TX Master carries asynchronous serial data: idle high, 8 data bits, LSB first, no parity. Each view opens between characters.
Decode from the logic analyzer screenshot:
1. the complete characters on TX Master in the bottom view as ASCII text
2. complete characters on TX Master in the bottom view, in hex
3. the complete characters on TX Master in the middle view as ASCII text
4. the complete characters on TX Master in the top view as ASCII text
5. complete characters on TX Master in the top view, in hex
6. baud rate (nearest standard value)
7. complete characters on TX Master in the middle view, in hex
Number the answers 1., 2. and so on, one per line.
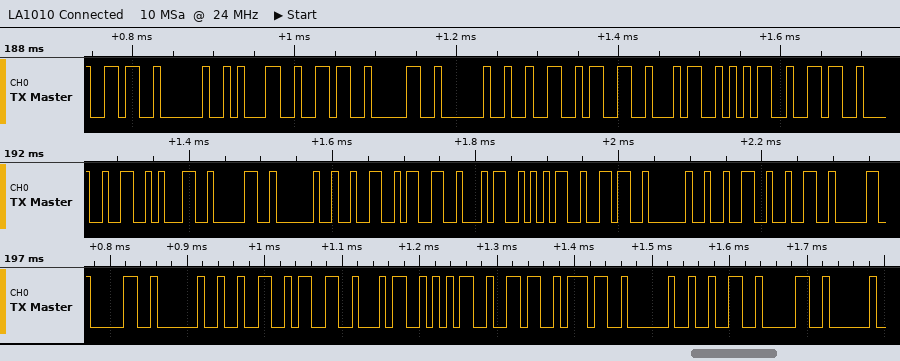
1. "0 234567 20"
2. 30, 20, 32, 33, 34, 35, 36, 37, 20, 32, 30
3. "210 23456 22"
4. "6 160 23456"
5. 36, 20, 31, 36, 30, 20, 32, 33, 34, 35, 36
6. 115200 baud
7. 32, 31, 30, 20, 32, 33, 34, 35, 36, 20, 32, 32
